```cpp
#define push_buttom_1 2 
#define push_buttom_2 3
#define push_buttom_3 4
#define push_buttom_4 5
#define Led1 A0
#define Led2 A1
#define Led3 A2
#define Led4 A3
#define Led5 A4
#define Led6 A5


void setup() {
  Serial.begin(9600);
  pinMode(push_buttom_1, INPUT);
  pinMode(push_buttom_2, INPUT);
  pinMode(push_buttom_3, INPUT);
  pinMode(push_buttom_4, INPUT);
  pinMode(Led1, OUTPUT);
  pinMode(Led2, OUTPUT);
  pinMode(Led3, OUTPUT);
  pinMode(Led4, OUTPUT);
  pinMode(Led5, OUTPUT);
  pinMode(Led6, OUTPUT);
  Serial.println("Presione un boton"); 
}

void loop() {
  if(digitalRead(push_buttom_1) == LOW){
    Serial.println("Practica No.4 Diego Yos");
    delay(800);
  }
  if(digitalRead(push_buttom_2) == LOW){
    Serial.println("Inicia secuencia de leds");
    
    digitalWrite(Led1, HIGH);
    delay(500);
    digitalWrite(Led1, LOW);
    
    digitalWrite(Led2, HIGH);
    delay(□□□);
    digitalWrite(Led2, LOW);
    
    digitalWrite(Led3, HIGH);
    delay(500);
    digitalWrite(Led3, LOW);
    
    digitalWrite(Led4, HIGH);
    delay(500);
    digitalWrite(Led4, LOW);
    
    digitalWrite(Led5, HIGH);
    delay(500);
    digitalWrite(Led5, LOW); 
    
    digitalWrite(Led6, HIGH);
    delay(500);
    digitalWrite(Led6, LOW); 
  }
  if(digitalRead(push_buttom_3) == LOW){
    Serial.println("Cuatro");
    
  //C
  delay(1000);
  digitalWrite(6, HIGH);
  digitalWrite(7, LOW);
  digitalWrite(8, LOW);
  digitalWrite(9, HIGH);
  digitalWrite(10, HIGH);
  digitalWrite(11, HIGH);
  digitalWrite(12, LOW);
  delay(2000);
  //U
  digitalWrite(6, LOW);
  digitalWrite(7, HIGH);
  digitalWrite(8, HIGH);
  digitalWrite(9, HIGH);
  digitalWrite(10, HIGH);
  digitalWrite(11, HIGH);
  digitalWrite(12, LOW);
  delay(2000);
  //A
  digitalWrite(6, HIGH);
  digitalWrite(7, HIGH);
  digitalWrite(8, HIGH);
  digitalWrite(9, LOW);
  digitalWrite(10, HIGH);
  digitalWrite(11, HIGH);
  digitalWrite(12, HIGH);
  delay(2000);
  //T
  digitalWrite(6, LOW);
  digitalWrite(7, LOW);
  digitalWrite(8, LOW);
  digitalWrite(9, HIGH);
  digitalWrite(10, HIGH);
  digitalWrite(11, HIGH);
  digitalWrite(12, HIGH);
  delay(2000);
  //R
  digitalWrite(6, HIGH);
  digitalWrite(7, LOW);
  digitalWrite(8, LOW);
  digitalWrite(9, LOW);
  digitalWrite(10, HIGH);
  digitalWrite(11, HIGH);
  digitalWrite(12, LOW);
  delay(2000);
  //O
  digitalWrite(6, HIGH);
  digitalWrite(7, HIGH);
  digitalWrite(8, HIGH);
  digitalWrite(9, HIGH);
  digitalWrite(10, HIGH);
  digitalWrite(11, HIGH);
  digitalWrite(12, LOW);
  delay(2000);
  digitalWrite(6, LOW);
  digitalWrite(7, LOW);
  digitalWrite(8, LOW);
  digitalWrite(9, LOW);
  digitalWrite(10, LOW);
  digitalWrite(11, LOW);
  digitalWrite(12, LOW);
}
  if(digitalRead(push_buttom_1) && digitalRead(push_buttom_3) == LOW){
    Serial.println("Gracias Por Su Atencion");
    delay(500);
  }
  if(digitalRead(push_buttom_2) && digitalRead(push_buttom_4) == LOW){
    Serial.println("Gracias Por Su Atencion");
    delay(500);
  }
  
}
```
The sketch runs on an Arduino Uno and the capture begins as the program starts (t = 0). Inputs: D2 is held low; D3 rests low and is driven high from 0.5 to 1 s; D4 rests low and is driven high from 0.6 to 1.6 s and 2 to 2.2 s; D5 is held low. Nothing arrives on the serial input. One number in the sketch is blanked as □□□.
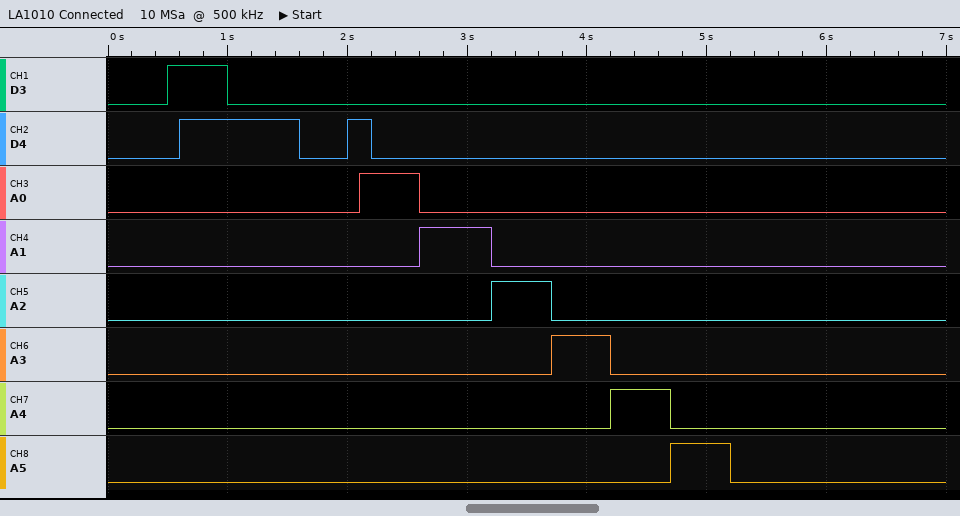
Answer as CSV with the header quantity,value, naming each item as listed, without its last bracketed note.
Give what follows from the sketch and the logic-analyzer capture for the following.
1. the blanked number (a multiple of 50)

quantity,value
the blanked number,600
